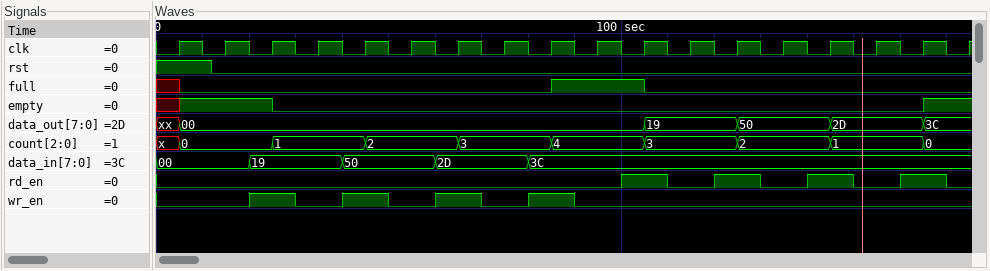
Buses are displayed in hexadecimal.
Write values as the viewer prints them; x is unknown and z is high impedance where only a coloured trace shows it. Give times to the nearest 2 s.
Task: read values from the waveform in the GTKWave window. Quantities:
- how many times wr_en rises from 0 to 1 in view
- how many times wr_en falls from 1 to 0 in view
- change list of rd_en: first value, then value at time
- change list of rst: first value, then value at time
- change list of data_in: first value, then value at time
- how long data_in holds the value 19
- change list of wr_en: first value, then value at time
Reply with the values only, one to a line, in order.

4
4
0, 1 at 100 s, 0 at 110 s, 1 at 120 s, 0 at 130 s, 1 at 140 s, 0 at 150 s, 1 at 160 s, 0 at 170 s
1, 0 at 12 s
00, 19 at 20 s, 50 at 40 s, 2D at 60 s, 3C at 80 s
20 s
0, 1 at 20 s, 0 at 30 s, 1 at 40 s, 0 at 50 s, 1 at 60 s, 0 at 70 s, 1 at 80 s, 0 at 90 s
